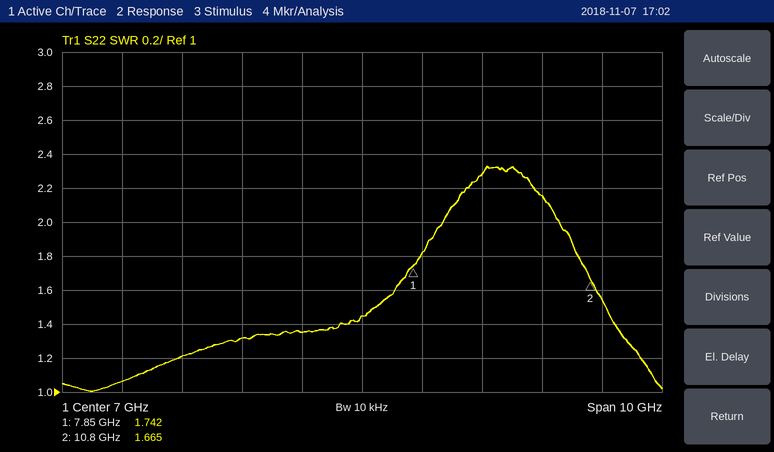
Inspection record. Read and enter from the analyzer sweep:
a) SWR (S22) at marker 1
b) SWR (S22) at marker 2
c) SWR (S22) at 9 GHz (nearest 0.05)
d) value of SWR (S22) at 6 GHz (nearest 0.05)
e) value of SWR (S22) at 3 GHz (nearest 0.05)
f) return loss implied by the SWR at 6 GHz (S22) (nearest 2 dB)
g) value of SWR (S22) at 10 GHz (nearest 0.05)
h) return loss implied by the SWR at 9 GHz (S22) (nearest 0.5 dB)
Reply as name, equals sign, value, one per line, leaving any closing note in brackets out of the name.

SWR (S22) at marker 1 = 1.742
SWR (S22) at marker 2 = 1.665
SWR (S22) at 9 GHz = 2.30
value of SWR (S22) at 6 GHz = 1.35
value of SWR (S22) at 3 GHz = 1.05
return loss implied by the SWR at 6 GHz (S22) = 16 dB
value of SWR (S22) at 10 GHz = 2.15
return loss implied by the SWR at 9 GHz (S22) = 8.0 dB
